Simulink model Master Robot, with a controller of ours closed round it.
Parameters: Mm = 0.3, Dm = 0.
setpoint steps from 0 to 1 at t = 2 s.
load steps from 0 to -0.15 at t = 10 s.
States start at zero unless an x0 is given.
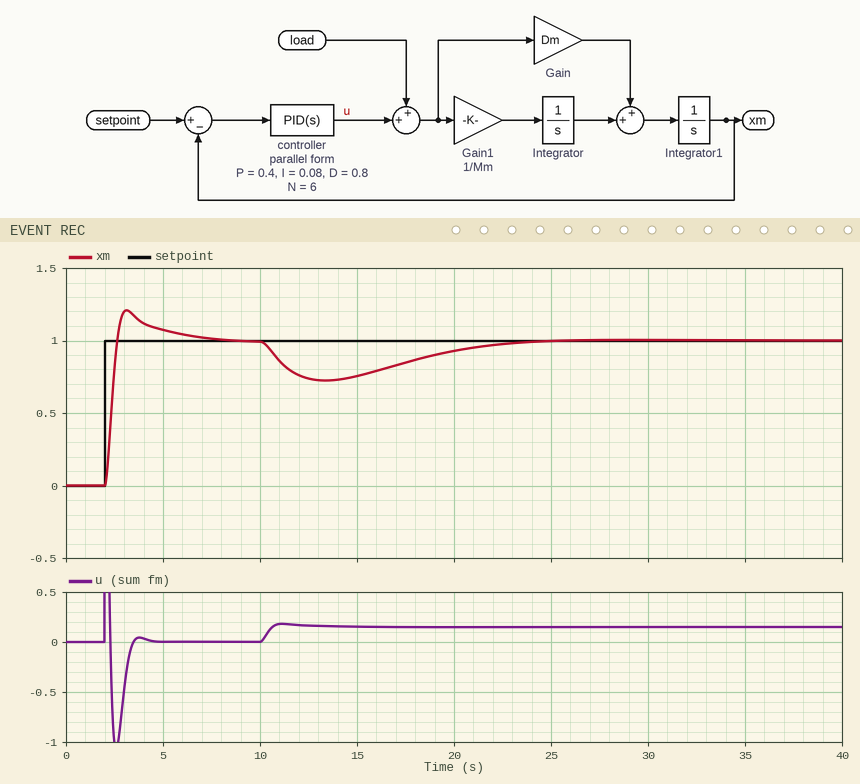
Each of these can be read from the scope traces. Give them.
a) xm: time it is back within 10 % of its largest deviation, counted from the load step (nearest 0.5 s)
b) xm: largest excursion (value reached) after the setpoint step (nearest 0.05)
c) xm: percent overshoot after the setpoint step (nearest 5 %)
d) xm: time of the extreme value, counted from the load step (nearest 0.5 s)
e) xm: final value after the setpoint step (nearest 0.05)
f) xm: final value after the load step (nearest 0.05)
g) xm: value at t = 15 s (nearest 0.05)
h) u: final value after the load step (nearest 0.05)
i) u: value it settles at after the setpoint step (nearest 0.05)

12.5 s
1.20
20 %
3.5 s
1.00
1.00
0.75
0.15
0.00
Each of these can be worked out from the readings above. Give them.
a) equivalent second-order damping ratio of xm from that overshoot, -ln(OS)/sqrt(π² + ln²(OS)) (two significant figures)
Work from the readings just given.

0.46
